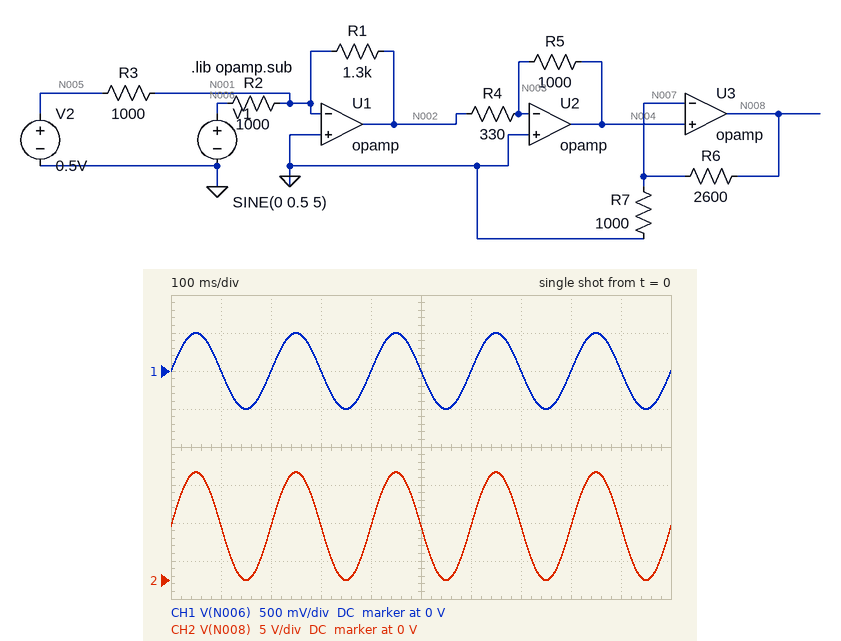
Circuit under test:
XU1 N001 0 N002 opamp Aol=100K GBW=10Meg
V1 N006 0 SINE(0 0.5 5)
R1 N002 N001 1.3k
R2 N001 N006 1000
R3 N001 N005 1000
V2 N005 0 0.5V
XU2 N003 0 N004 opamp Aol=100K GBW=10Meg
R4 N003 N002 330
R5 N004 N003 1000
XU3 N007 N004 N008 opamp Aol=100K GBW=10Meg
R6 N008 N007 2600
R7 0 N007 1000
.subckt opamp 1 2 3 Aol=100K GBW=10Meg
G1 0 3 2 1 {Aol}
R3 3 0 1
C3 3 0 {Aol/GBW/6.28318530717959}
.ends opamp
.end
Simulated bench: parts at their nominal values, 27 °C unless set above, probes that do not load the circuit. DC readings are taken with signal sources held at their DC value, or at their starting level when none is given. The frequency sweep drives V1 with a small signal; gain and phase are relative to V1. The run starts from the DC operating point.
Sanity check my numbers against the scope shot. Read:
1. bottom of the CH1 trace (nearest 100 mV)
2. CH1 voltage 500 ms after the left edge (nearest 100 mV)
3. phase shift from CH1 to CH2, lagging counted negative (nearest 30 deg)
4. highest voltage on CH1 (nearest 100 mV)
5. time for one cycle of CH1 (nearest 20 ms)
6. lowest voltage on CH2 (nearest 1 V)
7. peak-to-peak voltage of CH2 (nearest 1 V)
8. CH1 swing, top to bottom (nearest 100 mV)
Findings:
-500 mV
0 V
0 deg
500 mV
200 ms
0 V
14 V
1.0 V
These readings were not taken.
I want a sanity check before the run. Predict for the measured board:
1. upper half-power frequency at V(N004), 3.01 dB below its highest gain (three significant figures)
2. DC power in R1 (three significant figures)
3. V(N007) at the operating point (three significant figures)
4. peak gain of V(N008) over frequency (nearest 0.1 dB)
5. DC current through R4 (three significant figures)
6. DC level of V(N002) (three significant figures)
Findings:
1.69 MHz
325 µW
1.97 V
23.0 dB
1.97 mA
-650 mV
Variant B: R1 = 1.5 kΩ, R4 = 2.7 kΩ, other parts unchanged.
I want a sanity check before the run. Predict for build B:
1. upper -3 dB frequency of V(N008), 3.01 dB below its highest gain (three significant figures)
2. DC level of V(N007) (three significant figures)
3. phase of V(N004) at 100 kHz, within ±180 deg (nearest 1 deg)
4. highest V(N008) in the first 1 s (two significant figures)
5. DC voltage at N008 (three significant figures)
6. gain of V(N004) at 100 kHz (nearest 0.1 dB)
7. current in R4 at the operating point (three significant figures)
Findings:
1.62 MHz
278 mV
-3 deg
2.0 V
1.00 V
-5.1 dB
278 µA
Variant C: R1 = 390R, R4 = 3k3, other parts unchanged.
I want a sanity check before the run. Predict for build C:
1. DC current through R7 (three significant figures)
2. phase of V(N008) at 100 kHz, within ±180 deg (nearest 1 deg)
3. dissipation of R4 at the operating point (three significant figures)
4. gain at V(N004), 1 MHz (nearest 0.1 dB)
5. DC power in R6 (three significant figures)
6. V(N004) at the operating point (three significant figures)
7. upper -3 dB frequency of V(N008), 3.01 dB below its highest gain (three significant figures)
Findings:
59.1 µA
-4 deg
11.5 µW
-18.8 dB
9.08 µW
59.1 mV
2.17 MHz
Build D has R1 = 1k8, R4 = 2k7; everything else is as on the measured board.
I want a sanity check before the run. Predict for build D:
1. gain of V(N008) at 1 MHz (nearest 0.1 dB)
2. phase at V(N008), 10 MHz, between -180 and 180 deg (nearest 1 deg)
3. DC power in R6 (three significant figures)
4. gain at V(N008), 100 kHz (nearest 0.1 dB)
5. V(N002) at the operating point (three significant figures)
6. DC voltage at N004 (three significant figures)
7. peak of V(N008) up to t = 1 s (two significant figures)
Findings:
6.2 dB
154 deg
289 µW
7.6 dB
-900 mV
333 mV
2.4 V
